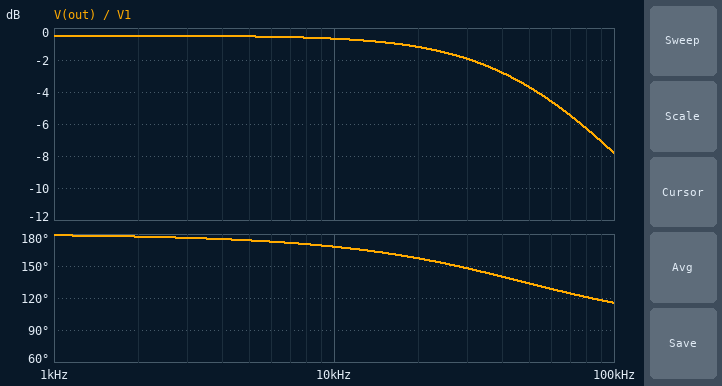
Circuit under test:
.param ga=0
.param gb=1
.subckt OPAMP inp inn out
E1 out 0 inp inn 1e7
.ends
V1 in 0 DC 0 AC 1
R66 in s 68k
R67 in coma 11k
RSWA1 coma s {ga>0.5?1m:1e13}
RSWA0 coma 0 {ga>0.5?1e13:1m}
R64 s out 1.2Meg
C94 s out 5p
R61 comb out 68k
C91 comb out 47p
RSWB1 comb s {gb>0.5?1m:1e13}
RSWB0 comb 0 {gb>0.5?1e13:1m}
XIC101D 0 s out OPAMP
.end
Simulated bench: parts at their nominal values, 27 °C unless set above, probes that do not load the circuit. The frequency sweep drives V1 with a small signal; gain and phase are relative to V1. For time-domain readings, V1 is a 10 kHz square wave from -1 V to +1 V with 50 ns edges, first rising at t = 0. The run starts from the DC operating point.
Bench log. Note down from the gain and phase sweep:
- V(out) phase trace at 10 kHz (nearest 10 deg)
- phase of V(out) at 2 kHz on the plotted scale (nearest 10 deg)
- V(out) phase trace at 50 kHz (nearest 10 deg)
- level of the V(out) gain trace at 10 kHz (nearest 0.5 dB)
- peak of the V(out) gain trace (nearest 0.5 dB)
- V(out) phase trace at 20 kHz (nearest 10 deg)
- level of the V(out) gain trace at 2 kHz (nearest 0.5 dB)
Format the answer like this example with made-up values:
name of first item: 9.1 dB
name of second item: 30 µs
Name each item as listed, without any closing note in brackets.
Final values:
V(out) phase trace at 10 kHz: 170 deg
phase of V(out) at 2 kHz on the plotted scale: 180 deg
V(out) phase trace at 50 kHz: 130 deg
level of the V(out) gain trace at 10 kHz: -0.5 dB
peak of the V(out) gain trace: -0.5 dB
V(out) phase trace at 20 kHz: 160 deg
level of the V(out) gain trace at 2 kHz: -0.5 dB
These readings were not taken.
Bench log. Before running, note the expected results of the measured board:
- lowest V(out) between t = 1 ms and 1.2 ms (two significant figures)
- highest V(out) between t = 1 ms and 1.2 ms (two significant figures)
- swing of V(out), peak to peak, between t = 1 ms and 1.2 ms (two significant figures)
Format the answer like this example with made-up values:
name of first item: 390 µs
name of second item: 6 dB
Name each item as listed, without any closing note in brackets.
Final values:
lowest V(out) between t = 1 ms and 1.2 ms: -950 mV
highest V(out) between t = 1 ms and 1.2 ms: 950 mV
swing of V(out), peak to peak, between t = 1 ms and 1.2 ms: 1.9 V
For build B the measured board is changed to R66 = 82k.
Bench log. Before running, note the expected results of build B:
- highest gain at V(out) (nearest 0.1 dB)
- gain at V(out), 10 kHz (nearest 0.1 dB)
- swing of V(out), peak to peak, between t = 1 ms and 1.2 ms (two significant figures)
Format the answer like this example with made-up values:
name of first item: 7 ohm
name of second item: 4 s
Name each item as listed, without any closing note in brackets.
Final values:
highest gain at V(out): -2.1 dB
gain at V(out), 10 kHz: -2.3 dB
swing of V(out), peak to peak, between t = 1 ms and 1.2 ms: 1.6 V
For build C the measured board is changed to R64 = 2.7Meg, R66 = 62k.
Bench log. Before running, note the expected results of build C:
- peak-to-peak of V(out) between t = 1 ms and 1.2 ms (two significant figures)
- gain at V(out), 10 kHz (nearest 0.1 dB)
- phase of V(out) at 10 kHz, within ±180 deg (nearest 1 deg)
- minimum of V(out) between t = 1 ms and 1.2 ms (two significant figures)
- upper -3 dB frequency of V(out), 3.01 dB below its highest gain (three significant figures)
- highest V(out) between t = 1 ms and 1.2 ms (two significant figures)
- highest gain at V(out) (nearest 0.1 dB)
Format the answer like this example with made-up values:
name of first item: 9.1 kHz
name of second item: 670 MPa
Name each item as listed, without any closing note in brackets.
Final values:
peak-to-peak of V(out) between t = 1 ms and 1.2 ms: 2.1 V
gain at V(out), 10 kHz: 0.4 dB
phase of V(out) at 10 kHz, within ±180 deg: 168 deg
minimum of V(out) between t = 1 ms and 1.2 ms: -1.1 V
upper -3 dB frequency of V(out), 3.01 dB below its highest gain: 46.1 kHz
highest V(out) between t = 1 ms and 1.2 ms: 1.1 V
highest gain at V(out): 0.6 dB
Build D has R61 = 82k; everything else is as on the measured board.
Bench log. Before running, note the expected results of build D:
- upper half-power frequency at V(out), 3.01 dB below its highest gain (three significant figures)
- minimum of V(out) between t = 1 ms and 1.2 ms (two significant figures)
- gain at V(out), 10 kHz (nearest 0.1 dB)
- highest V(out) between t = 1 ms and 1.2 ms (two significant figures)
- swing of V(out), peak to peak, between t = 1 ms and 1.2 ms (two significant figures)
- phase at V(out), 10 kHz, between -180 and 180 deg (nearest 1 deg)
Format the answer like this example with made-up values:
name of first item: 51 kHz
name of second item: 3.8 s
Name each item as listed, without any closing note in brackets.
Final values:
upper half-power frequency at V(out), 3.01 dB below its highest gain: 39.9 kHz
minimum of V(out) between t = 1 ms and 1.2 ms: -1.1 V
gain at V(out), 10 kHz: 0.8 dB
highest V(out) between t = 1 ms and 1.2 ms: 1.1 V
swing of V(out), peak to peak, between t = 1 ms and 1.2 ms: 2.3 V
phase at V(out), 10 kHz, between -180 and 180 deg: 166 deg
